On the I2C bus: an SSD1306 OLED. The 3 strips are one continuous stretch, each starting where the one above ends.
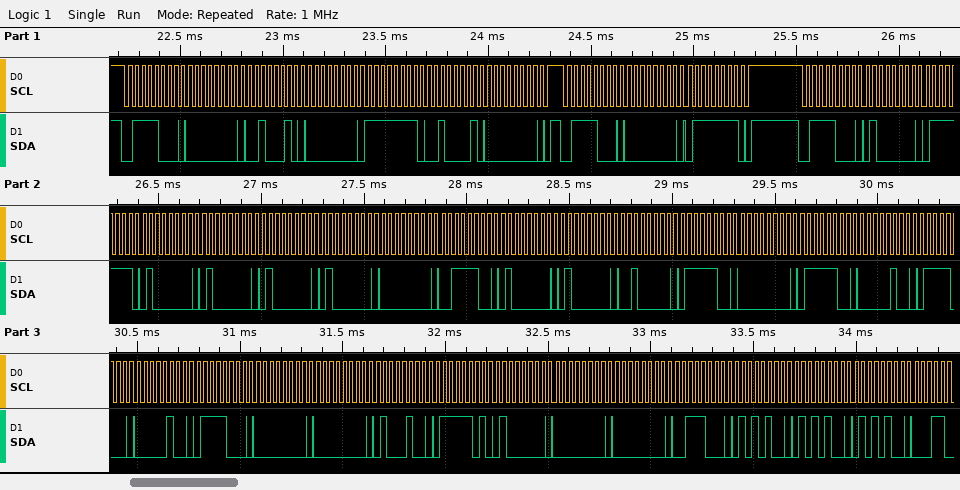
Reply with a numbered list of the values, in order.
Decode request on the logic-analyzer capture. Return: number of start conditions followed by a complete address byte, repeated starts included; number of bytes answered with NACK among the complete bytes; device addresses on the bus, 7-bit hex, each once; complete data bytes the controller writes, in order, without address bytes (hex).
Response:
1. 3
2. 0
3. 0x3C
4. 00 22 00 FF 21 00 00 7F 40 7F 40 40 40 40 00 3C 40 40 20 7C 00 7C 04 78 04 78 00 00 44 7D 40 00 00 38 54 54 54
